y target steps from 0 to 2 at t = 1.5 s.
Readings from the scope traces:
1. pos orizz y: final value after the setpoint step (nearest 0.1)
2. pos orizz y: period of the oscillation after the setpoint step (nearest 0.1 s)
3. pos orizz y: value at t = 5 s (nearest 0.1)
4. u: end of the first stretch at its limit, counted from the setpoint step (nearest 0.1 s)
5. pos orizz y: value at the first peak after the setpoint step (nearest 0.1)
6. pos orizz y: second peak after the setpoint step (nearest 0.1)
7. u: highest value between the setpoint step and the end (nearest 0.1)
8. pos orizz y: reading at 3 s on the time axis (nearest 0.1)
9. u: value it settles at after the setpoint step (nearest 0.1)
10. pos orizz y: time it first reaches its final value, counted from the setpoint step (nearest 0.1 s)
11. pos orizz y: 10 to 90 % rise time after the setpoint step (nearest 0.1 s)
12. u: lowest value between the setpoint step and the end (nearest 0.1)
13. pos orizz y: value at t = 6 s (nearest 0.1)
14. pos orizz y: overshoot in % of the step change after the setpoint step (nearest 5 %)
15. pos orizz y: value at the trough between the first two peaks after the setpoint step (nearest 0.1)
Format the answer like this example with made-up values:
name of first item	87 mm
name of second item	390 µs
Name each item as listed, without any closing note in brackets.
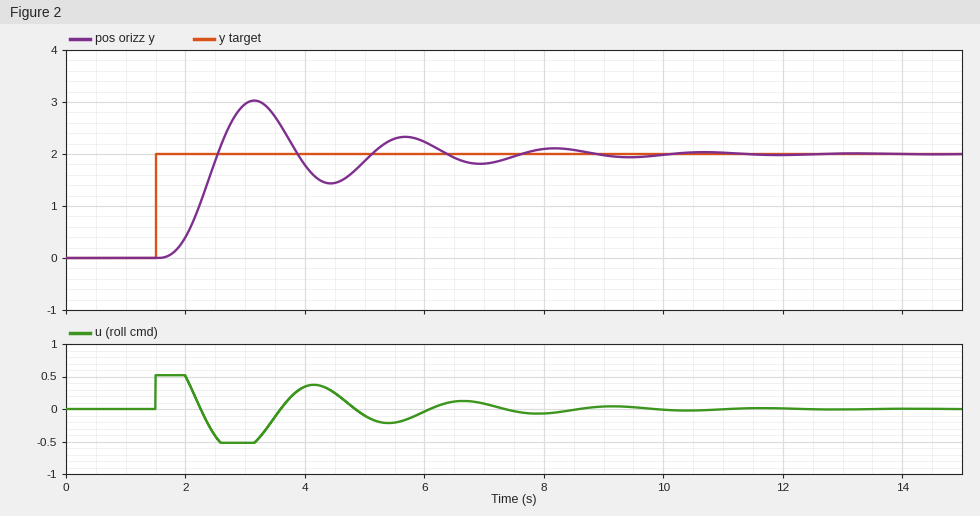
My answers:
pos orizz y: final value after the setpoint step	2.0
pos orizz y: period of the oscillation after the setpoint step	2.5 s
pos orizz y: value at t = 5 s	1.9
u: end of the first stretch at its limit, counted from the setpoint step	0.5 s
pos orizz y: value at the first peak after the setpoint step	3.0
pos orizz y: second peak after the setpoint step	2.3
u: highest value between the setpoint step and the end	0.5
pos orizz y: reading at 3 s on the time axis	3.0
u: value it settles at after the setpoint step	0.0
pos orizz y: time it first reaches its final value, counted from the setpoint step	1.0 s
pos orizz y: 10 to 90 % rise time after the setpoint step	0.6 s
u: lowest value between the setpoint step and the end	-0.5
pos orizz y: value at t = 6 s	2.2
pos orizz y: overshoot in % of the step change after the setpoint step	50 %
pos orizz y: value at the trough between the first two peaks after the setpoint step	1.4
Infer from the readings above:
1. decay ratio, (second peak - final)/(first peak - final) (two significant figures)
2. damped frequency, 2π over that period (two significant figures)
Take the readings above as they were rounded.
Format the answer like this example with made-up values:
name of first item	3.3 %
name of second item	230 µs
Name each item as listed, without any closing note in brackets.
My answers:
decay ratio, (second peak - final)/(first peak - final)	0.30
damped frequency, 2π over that period	2.5 rad/s
